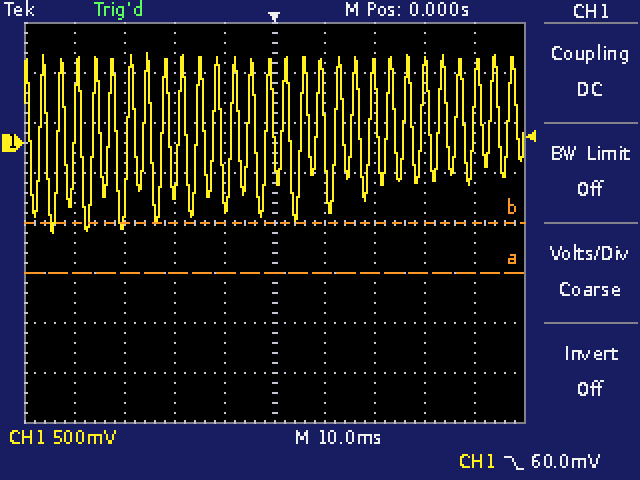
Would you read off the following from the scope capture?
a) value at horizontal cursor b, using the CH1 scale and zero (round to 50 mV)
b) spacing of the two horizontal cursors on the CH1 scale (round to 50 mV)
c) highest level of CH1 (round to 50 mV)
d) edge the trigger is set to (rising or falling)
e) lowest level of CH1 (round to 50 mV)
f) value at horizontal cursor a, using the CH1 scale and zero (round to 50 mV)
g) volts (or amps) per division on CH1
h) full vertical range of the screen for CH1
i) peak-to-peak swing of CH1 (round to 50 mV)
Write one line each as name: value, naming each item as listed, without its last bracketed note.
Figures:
value at horizontal cursor b, using the CH1 scale and zero: -800 mV
spacing of the two horizontal cursors on the CH1 scale: 500 mV
highest level of CH1: 900 mV
edge the trigger is set to: falling
lowest level of CH1: -900 mV
value at horizontal cursor a, using the CH1 scale and zero: -1.30 V
volts (or amps) per division on CH1: 500 mV
full vertical range of the screen for CH1: 4 V
peak-to-peak swing of CH1: 1.80 V
